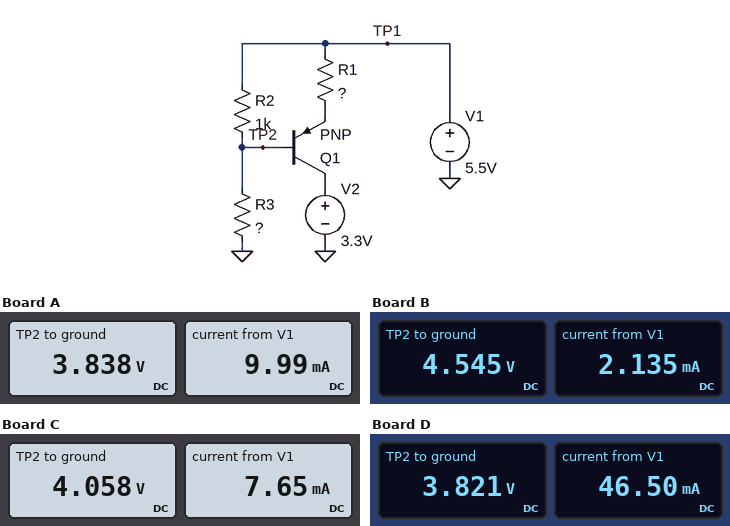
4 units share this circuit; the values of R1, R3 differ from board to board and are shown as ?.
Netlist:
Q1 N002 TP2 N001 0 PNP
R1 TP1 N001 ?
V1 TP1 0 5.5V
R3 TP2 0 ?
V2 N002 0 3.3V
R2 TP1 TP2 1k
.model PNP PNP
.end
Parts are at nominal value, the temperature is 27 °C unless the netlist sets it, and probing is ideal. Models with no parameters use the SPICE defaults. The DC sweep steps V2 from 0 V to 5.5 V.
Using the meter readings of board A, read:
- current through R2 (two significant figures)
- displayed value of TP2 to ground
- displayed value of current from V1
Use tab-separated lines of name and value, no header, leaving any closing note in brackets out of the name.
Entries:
current through R2	1.7 mA
displayed value of TP2 to ground	3.838 V
displayed value of current from V1	9.99 mA
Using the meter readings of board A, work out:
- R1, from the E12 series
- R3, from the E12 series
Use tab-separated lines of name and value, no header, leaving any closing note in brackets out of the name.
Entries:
R1, from the E12 series	100 Ω
R3, from the E12 series	2.2 kΩ
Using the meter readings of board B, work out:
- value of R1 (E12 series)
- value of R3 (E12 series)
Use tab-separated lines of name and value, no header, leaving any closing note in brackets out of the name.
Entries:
value of R1	150 Ω
value of R3	4.7 kΩ
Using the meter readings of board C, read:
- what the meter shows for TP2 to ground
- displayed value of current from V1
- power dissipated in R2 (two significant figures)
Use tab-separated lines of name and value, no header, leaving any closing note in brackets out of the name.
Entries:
what the meter shows for TP2 to ground	4.058 V
displayed value of current from V1	7.65 mA
power dissipated in R2	2.1 mW
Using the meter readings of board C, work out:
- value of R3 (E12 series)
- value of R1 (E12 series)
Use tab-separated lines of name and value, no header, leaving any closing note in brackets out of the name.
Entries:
value of R3	2.7 kΩ
value of R1	100 Ω
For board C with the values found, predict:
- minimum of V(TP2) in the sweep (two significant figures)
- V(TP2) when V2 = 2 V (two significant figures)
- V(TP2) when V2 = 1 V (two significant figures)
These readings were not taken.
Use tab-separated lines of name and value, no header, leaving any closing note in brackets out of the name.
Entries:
minimum of V(TP2) in the sweep	4.1 V
V(TP2) when V2 = 2 V	4.1 V
V(TP2) when V2 = 1 V	4.1 V
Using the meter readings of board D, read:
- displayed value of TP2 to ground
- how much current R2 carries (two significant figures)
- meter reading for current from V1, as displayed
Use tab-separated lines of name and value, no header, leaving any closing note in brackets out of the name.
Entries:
displayed value of TP2 to ground	3.821 V
how much current R2 carries	1.7 mA
meter reading for current from V1, as displayed	46.50 mA
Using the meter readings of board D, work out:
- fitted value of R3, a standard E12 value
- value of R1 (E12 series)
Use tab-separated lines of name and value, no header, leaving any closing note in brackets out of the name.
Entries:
fitted value of R3, a standard E12 value	1.8 kΩ
value of R1	18 Ω
